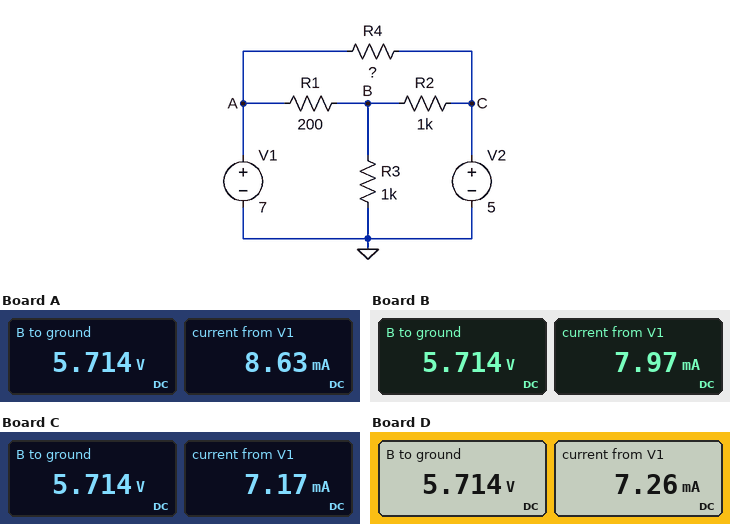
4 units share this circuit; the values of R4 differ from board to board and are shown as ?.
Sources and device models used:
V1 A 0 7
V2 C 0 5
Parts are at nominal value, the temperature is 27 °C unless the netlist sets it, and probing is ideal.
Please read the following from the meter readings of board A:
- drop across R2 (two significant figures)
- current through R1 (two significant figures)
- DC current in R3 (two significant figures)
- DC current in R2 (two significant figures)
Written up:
710 mV
6.4 mA
5.7 mA
710 µA
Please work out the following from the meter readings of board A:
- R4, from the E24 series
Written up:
910 Ω
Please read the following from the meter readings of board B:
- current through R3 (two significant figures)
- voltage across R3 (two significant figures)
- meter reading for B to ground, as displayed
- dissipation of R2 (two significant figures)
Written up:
5.7 mA
5.7 V
5.714 V
510 µW
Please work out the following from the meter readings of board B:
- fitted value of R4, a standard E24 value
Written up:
1.3 kΩ
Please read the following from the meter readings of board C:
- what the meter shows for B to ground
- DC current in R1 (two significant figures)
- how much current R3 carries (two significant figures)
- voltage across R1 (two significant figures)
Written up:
5.714 V
6.4 mA
5.7 mA
1.3 V
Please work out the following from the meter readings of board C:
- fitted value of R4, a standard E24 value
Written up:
2.7 kΩ
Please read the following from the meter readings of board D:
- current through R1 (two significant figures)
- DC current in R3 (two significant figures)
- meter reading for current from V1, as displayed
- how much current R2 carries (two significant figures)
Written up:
6.4 mA
5.7 mA
7.26 mA
710 µA
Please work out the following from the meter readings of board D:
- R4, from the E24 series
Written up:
2.4 kΩ
